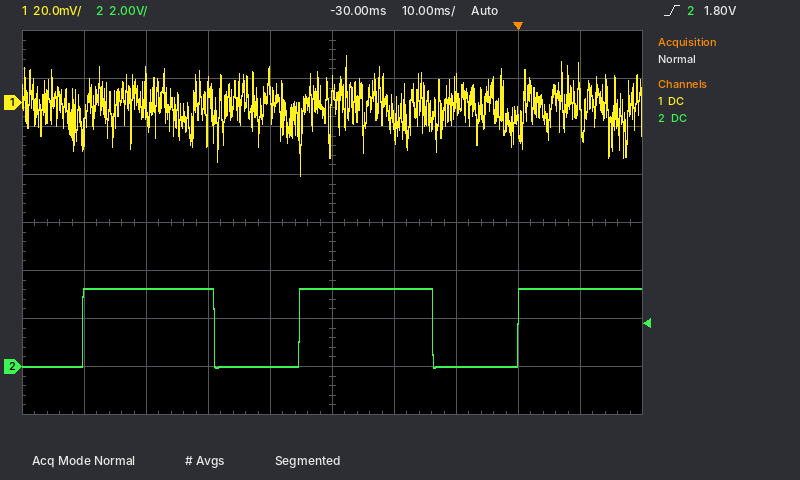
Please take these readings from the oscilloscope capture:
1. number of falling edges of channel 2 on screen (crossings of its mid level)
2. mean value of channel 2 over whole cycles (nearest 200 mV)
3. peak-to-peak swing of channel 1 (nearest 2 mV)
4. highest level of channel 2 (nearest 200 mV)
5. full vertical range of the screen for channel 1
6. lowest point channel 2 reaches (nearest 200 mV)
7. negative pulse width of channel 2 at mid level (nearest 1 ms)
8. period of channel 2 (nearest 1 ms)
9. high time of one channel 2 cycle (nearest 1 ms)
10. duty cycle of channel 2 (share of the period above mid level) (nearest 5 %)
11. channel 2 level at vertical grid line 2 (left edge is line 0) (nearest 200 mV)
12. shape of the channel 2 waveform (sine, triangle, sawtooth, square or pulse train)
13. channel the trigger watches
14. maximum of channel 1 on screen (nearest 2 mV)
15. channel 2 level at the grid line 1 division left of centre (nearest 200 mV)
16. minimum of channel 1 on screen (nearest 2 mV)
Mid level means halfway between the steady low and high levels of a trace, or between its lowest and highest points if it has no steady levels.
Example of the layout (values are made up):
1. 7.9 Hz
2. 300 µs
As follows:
1. 2
2. 2.0 V
3. 50 mV
4. 3.2 V
5. 160 mV
6. 0.0 V
7. 14 ms
8. 35 ms
9. 21 ms
10. 60 %
11. 3.2 V
12. pulse train
13. channel 2
14. 20 mV
15. 0.0 V
16. -30 mV
